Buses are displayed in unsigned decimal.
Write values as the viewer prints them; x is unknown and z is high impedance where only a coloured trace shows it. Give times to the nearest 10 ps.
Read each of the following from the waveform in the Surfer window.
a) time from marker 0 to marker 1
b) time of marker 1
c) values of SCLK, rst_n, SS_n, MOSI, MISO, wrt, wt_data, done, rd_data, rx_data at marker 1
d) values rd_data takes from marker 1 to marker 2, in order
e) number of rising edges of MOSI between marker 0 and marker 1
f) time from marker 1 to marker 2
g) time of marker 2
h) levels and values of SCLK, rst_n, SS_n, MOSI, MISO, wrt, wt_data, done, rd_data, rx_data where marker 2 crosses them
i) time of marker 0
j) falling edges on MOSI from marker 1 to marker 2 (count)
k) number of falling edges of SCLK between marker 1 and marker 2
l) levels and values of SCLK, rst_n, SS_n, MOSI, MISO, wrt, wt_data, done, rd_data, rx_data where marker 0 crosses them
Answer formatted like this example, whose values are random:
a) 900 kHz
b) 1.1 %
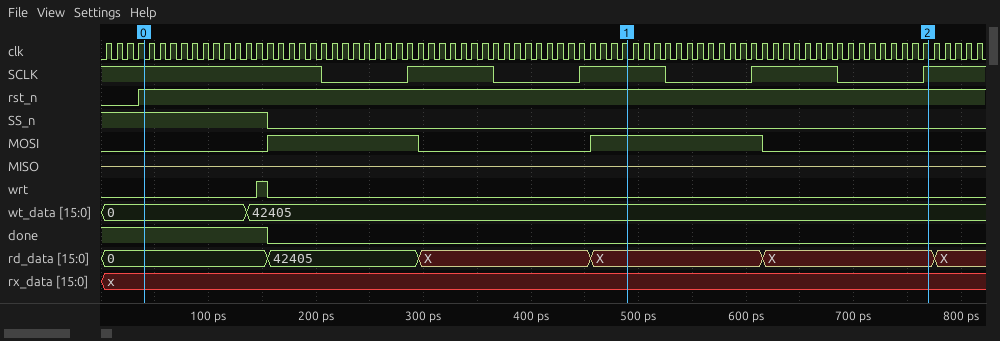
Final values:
a) 450 ps
b) 490 ps
c) SCLK=1, rst_n=1, SS_n=0, MOSI=1, MISO=z, wrt=0, wt_data=42405, done=0, rd_data=X, rx_data=x
d) X, X
e) 2
f) 280 ps
g) 770 ps
h) SCLK=1, rst_n=1, SS_n=0, MOSI=0, MISO=z, wrt=0, wt_data=42405, done=0, rd_data=X, rx_data=x
i) 40 ps
j) 1
k) 2
l) SCLK=1, rst_n=1, SS_n=1, MOSI=0, MISO=z, wrt=0, wt_data=0, done=1, rd_data=0, rx_data=x
